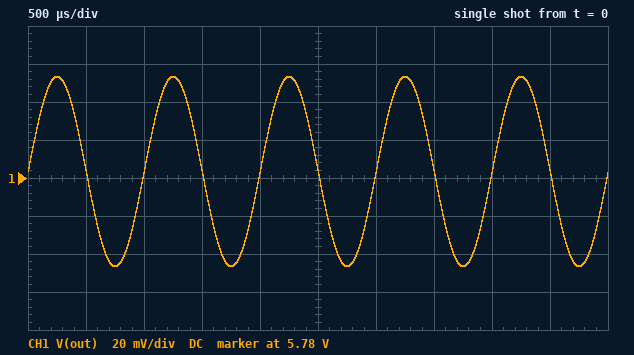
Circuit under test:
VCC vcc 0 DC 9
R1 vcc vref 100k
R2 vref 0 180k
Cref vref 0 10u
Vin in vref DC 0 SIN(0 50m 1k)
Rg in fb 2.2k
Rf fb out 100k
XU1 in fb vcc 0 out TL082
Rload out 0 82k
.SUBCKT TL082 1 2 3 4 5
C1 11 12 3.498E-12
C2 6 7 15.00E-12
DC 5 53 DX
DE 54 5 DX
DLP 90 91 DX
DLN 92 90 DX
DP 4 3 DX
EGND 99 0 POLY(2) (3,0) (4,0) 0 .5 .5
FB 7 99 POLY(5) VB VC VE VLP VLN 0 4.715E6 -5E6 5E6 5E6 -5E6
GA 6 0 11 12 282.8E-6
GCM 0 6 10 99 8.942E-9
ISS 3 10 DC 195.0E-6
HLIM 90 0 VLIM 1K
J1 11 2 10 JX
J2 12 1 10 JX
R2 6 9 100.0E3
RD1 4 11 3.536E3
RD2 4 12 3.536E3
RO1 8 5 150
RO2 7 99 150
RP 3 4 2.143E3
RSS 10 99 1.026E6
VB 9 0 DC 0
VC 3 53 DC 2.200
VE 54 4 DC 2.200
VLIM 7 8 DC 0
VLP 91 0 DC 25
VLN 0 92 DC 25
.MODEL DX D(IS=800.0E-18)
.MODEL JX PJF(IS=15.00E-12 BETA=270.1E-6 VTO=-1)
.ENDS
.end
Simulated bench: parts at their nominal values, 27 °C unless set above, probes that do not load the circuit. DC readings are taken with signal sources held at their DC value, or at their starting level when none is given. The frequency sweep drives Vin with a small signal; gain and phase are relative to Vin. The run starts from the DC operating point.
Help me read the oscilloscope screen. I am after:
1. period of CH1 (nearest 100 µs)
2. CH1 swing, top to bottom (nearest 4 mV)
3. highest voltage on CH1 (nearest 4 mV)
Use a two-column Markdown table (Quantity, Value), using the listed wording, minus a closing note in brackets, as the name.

| Quantity | Value |
|---|---|
| period of CH1 | 1.0 ms |
| CH1 swing, top to bottom | 100 mV |
| highest voltage on CH1 | 5.832 V |
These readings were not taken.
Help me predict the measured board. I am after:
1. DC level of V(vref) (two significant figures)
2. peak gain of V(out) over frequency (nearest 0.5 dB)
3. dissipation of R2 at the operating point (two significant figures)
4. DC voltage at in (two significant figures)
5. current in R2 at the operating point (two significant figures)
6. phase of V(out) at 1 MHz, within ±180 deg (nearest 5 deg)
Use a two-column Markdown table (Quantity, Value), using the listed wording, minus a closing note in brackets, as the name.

| Quantity | Value |
|---|---|
| DC level of V(vref) | 5.8 V |
| peak gain of V(out) over frequency | 0 dB |
| dissipation of R2 at the operating point | 190 µW |
| DC voltage at in | 5.8 V |
| current in R2 at the operating point | 32 µA |
| phase of V(out) at 1 MHz, within ±180 deg | -95 deg |
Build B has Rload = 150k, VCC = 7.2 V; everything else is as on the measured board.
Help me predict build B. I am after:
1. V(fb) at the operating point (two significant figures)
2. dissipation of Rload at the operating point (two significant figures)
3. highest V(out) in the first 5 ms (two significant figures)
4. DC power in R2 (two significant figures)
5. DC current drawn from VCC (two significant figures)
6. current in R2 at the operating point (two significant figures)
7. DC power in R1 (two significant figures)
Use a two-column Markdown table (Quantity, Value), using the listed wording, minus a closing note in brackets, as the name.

| Quantity | Value |
|---|---|
| V(fb) at the operating point | 4.6 V |
| dissipation of Rload at the operating point | 140 µW |
| highest V(out) in the first 5 ms | 4.7 V |
| DC power in R2 | 120 µW |
| DC current drawn from VCC | 3.6 mA |
| current in R2 at the operating point | 26 µA |
| DC power in R1 | 66 µW |
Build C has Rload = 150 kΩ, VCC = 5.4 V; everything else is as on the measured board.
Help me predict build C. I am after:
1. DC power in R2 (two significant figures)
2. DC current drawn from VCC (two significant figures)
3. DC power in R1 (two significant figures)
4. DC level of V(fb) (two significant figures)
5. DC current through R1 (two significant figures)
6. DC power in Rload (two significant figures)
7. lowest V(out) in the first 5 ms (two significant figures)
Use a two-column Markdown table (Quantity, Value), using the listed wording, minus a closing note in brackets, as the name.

| Quantity | Value |
|---|---|
| DC power in R2 | 67 µW |
| DC current drawn from VCC | 2.7 mA |
| DC power in R1 | 37 µW |
| DC level of V(fb) | 3.5 V |
| DC current through R1 | 19 µA |
| DC power in Rload | 80 µW |
| lowest V(out) in the first 5 ms | 3.4 V |
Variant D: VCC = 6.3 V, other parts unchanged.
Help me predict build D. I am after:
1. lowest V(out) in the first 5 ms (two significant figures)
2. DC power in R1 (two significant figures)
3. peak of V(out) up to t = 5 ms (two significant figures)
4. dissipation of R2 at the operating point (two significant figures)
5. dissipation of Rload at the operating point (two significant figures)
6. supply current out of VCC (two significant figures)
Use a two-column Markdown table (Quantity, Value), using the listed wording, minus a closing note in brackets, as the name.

| Quantity | Value |
|---|---|
| lowest V(out) in the first 5 ms | 4.0 V |
| DC power in R1 | 51 µW |
| peak of V(out) up to t = 5 ms | 4.1 V |
| dissipation of R2 at the operating point | 91 µW |
| dissipation of Rload at the operating point | 200 µW |
| supply current out of VCC | 3.2 mA |
